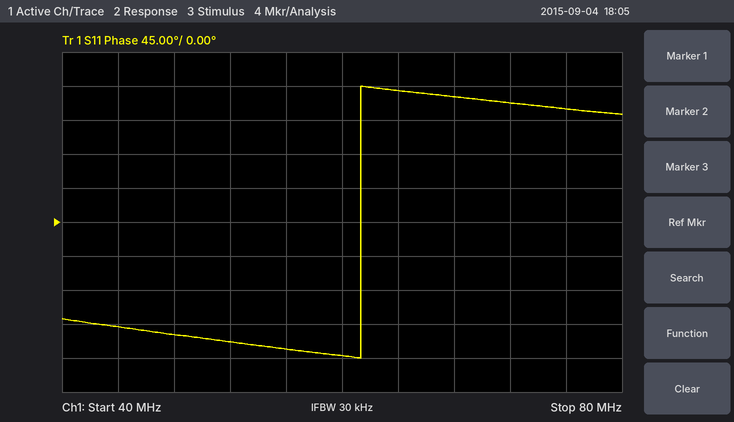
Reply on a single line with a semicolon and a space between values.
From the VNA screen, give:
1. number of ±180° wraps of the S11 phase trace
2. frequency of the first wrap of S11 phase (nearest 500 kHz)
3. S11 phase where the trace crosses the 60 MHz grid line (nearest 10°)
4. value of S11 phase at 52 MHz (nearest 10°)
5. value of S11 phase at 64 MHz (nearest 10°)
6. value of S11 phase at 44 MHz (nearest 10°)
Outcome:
1; 61.5 MHz; -180°; -160°; 170°; -140°
